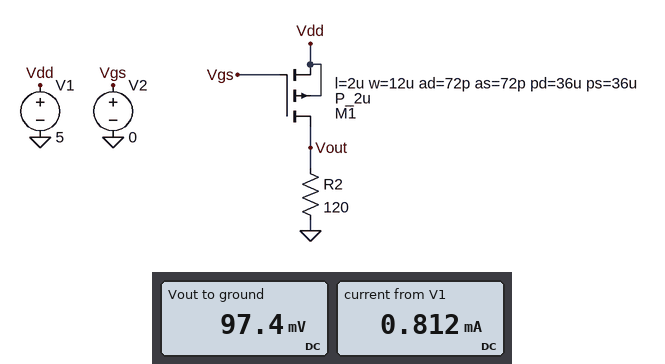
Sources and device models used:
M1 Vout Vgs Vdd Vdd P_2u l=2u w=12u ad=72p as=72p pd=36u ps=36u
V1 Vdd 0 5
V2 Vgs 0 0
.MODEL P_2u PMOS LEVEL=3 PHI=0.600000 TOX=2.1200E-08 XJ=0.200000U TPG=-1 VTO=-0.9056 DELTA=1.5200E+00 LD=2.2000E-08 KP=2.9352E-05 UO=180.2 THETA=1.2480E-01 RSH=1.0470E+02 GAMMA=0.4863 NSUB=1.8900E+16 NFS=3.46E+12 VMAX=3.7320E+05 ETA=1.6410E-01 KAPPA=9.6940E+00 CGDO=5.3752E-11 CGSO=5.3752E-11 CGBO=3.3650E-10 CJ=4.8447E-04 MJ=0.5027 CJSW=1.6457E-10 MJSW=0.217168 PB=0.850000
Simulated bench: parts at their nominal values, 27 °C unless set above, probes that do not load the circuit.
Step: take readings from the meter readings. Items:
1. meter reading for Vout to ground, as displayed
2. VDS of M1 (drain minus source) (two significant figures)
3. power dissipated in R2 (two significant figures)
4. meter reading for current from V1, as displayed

97.4 mV
-4.9 V
79 µW
0.812 mA
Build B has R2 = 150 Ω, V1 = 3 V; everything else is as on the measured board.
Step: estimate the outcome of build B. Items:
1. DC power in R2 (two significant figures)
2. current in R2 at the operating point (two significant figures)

11 µW
270 µA
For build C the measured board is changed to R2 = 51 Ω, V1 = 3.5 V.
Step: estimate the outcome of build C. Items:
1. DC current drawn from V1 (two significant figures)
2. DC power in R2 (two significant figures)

380 µA
7.5 µW
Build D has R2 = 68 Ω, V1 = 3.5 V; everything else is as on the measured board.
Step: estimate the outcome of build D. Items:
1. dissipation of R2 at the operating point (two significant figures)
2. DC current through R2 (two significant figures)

10 µW
380 µA
